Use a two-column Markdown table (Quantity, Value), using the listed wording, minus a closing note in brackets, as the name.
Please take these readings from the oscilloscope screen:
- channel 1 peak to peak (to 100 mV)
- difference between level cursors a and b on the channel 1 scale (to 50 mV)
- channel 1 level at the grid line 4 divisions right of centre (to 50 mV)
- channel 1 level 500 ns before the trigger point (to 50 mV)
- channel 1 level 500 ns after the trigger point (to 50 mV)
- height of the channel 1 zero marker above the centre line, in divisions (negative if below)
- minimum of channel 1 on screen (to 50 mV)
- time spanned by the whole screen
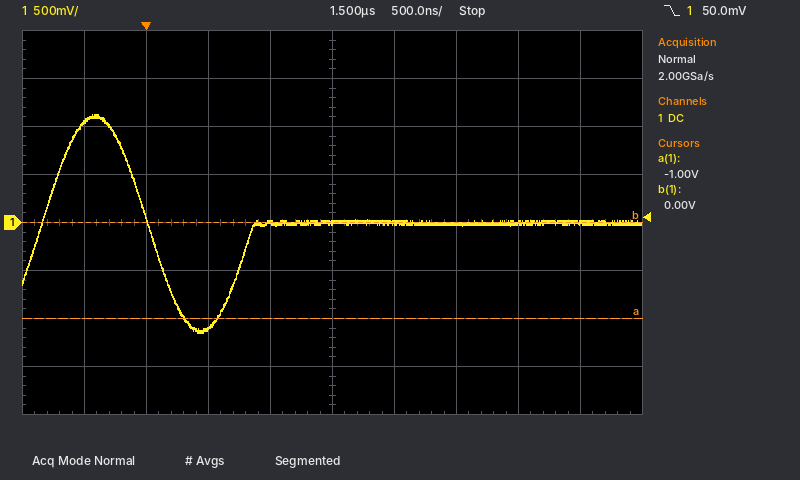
| Quantity | Value |
|---|---|
| channel 1 peak to peak | 2.30 V |
| difference between level cursors a and b on the channel 1 scale | 1.00 V |
| channel 1 level at the grid line 4 divisions right of centre | 0 mV |
| channel 1 level 500 ns before the trigger point | 1.05 V |
| channel 1 level 500 ns after the trigger point | -1.10 V |
| height of the channel 1 zero marker above the centre line, in divisions | 0.0 div |
| minimum of channel 1 on screen | -1.15 V |
| time spanned by the whole screen | 5 µs |
